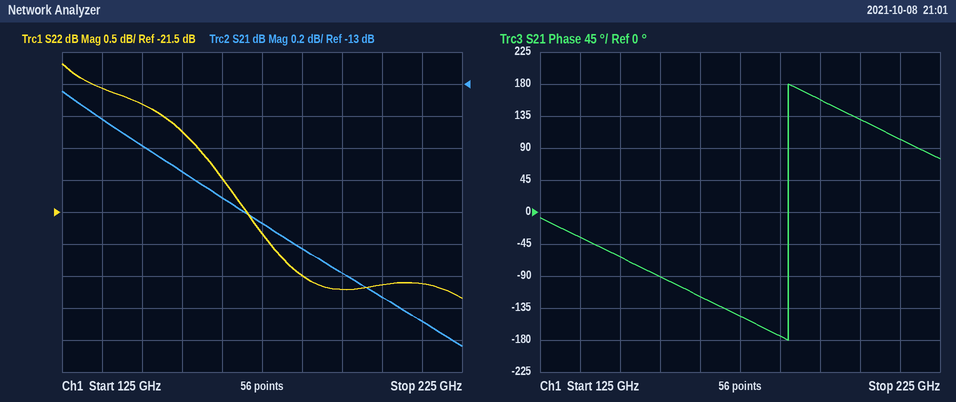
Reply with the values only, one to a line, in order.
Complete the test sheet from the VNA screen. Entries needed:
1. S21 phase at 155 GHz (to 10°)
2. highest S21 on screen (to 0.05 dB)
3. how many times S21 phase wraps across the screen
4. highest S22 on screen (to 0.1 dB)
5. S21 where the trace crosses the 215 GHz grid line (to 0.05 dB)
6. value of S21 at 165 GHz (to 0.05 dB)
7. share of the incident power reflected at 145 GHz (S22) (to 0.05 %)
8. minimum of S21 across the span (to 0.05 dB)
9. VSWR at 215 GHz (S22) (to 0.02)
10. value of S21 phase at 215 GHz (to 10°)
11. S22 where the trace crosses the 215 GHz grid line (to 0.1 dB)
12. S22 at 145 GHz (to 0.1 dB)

-90°
-13.05 dB
1
-19.2 dB
-14.50 dB
-13.70 dB
1.05 %
-14.65 dB
1.16
100°
-22.6 dB
-19.8 dB
